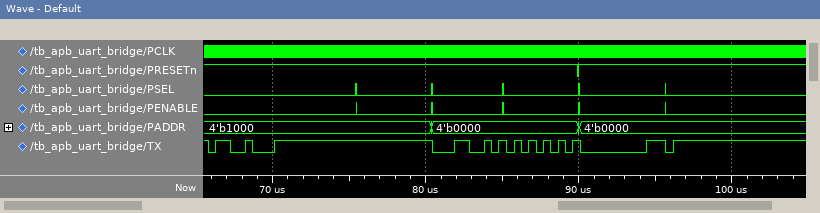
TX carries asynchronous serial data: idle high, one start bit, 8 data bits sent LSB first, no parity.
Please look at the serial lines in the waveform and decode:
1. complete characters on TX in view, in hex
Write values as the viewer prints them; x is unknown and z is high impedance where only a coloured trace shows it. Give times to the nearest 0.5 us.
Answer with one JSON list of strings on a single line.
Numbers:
["13, 4C, 55, 00, FF"]
